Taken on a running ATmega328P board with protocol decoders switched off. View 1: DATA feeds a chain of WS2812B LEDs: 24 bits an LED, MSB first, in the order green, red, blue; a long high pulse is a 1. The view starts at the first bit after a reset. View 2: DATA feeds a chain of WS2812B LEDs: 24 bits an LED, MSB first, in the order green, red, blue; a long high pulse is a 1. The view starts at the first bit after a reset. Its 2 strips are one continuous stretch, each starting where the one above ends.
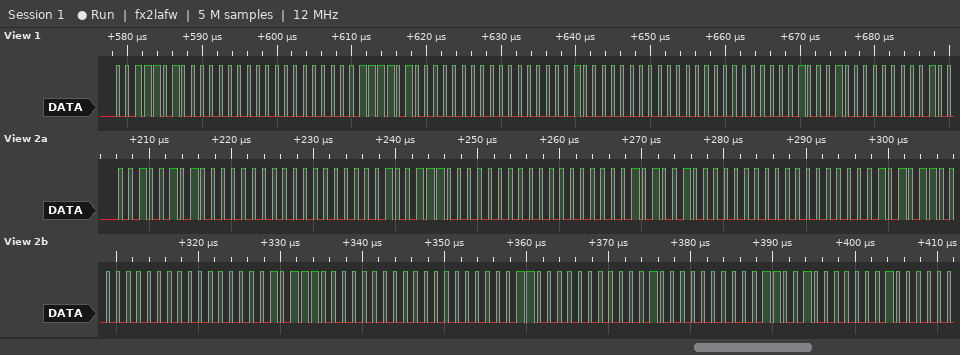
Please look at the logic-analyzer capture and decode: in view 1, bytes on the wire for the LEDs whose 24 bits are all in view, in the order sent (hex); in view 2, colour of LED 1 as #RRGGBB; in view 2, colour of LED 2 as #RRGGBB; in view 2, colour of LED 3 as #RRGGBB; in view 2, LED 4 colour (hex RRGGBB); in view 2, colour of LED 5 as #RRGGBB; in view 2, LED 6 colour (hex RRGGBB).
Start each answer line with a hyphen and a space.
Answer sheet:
- 3A 00 00 3D 00 00 40 00 00
- #002500
- #002700
- #002900
- #002B00
- #002E00
- #013000
